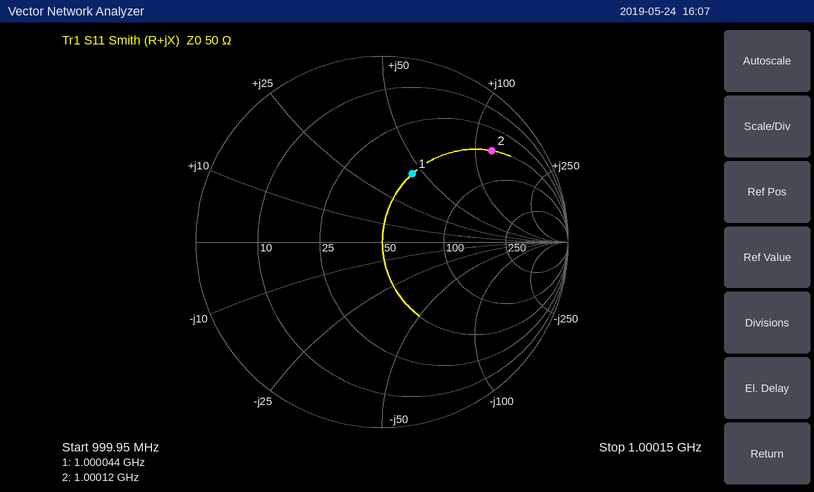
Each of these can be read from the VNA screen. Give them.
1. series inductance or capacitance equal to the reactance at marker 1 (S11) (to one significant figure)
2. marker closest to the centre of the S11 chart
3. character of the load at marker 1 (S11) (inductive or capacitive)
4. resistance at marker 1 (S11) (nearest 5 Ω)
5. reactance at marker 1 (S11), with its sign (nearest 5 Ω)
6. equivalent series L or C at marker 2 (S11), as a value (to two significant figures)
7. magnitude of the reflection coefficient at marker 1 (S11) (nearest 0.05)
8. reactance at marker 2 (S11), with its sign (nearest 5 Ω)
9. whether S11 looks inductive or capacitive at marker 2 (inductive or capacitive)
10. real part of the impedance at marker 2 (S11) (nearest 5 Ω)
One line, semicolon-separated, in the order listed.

7 nH; marker 1; inductive; 50 Ω; +45 Ω; 19 nH; 0.40; +120 Ω; inductive; 50 Ω
